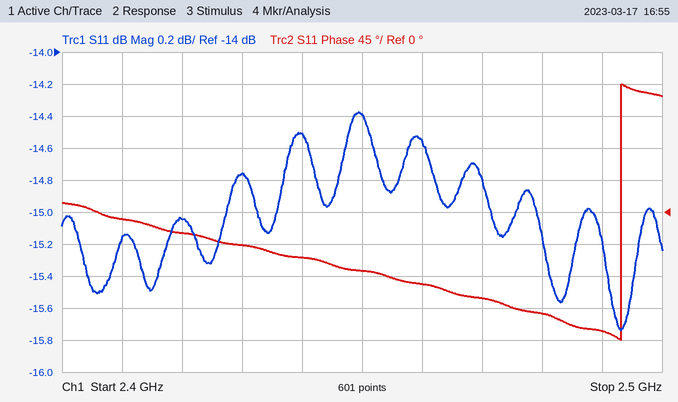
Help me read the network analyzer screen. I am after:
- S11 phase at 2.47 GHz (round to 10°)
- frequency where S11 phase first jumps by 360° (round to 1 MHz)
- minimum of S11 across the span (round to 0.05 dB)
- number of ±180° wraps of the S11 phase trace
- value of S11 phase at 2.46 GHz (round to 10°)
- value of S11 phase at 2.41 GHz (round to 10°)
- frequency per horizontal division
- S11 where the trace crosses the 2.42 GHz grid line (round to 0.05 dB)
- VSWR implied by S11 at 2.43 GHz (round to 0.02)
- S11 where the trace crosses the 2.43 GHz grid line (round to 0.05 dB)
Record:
-120°
2.493 GHz
-15.75 dB
1
-100°
-10°
10 MHz
-15.05 dB
1.44
-14.75 dB
